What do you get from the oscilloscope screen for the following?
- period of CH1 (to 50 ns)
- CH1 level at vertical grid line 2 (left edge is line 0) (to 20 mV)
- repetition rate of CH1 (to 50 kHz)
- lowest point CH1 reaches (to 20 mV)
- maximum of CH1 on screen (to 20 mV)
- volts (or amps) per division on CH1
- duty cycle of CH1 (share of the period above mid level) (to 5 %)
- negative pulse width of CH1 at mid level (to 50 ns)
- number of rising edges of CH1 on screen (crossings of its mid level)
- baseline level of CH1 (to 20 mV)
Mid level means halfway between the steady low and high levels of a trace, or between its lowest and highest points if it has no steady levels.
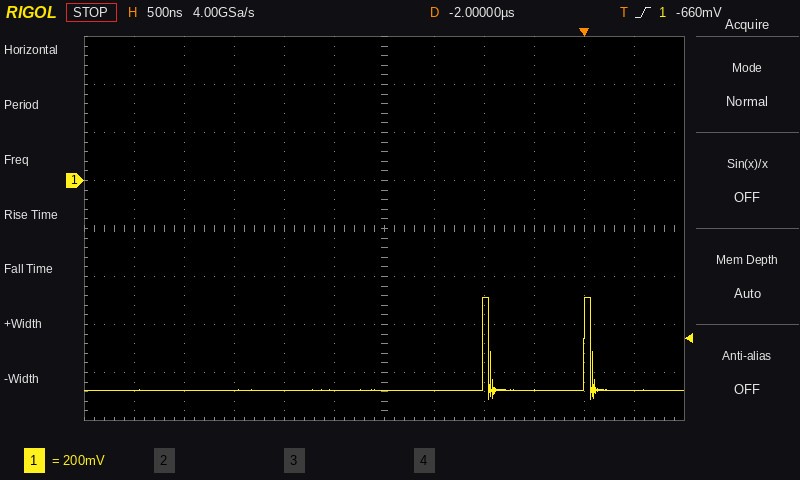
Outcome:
1.00 µs
-880 mV
1.00 MHz
-920 mV
-480 mV
200 mV
5 %
950 ns
2
-880 mV
